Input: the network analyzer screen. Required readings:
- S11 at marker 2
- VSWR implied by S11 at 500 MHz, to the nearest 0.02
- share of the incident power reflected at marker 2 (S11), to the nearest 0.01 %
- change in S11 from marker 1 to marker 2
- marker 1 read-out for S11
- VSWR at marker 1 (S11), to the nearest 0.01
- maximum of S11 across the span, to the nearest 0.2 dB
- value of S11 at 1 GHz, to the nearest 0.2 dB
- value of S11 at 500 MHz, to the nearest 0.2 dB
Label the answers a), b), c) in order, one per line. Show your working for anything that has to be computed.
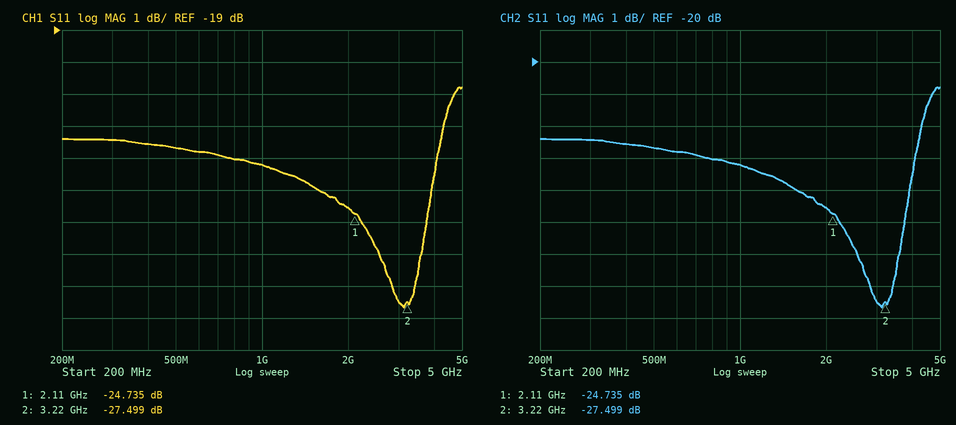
a) -27.499 dB
b) |Γ| = 10^(-22.6/20) = 0.0741; VSWR = (1 + 0.0741)/(1 − 0.0741) ≈ 1.16
c) 10^(-27.499/10) ≈ 0.18 %
d) -27.499 − (-24.735) = -2.764 dB
e) -24.735 dB
f) (1 + 0.0580)/(1 − 0.0580) ≈ 1.12
g) -20.8 dB
h) -23.2 dB
i) -22.6 dB
